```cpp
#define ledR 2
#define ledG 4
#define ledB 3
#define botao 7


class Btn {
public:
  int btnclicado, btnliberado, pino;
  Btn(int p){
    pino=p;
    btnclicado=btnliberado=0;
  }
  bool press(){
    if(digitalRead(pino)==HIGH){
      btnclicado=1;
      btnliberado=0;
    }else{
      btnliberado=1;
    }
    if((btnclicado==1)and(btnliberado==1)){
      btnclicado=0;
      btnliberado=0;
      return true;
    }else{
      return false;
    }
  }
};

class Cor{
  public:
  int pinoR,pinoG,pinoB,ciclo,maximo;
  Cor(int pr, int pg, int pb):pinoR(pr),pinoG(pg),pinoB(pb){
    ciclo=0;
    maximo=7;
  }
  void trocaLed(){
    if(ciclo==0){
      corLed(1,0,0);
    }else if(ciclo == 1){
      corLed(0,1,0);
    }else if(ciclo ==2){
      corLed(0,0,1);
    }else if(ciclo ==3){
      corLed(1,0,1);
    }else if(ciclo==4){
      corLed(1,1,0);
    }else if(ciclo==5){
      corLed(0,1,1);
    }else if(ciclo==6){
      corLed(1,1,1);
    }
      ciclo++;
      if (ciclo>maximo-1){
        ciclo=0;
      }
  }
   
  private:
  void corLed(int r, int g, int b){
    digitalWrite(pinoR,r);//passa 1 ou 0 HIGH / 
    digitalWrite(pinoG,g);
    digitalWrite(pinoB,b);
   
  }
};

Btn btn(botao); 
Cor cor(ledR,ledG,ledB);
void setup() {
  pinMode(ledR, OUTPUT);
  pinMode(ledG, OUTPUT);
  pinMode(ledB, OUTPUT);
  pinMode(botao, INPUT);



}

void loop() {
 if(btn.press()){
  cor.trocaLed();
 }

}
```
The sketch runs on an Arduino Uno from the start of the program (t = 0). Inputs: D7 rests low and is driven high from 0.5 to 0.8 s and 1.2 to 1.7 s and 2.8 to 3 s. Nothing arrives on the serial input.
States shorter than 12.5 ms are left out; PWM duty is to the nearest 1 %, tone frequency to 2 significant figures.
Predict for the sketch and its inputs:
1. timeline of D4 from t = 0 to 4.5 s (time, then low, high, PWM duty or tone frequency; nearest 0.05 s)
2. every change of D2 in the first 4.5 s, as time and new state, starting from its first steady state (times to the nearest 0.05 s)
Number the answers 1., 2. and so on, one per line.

1. 0 s low; 1.7 s high; 3 s low
2. 0 s low; 0.8 s high; 1.7 s low
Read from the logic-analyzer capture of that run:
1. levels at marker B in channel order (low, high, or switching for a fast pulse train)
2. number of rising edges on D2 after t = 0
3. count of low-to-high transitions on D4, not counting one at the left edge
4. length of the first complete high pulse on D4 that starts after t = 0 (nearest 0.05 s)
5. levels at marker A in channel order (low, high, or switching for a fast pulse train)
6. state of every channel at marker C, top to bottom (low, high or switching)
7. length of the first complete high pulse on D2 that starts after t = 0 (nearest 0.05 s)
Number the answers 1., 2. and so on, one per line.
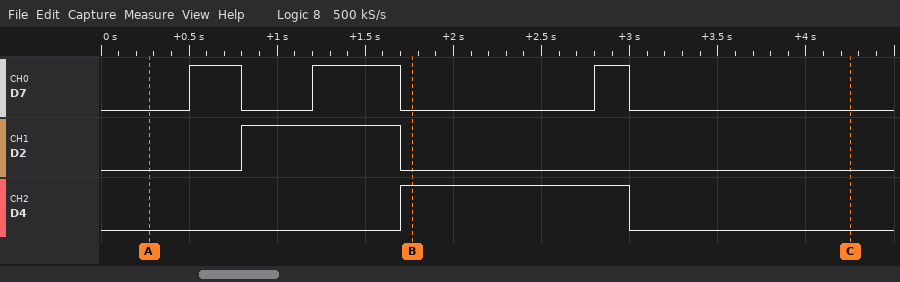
1. D7 low, D2 low, D4 high
2. 1
3. 1
4. 1.30 s
5. D7 low, D2 low, D4 low
6. D7 low, D2 low, D4 low
7. 0.90 s
